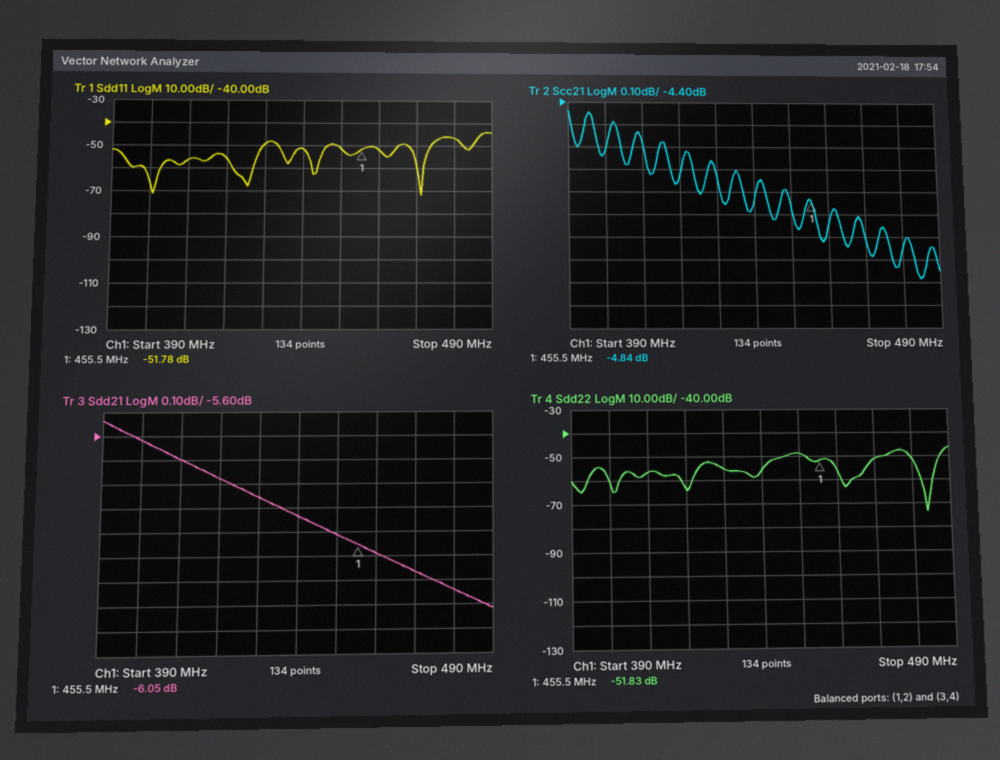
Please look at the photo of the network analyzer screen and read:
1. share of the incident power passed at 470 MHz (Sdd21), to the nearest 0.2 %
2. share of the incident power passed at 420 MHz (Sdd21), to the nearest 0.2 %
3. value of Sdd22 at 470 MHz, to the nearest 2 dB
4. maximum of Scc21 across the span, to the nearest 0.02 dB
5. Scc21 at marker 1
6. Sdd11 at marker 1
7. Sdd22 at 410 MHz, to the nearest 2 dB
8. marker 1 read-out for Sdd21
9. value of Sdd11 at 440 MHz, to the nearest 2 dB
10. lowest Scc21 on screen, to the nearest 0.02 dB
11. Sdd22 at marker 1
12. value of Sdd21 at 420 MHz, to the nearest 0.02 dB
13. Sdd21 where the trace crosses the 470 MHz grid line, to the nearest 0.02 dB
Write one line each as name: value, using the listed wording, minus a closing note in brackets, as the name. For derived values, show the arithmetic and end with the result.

share of the incident power passed at 470 MHz (Sdd21), to the nearest 0.2 %: 10^(-6.16/10) ≈ 24.2 %
share of the incident power passed at 420 MHz (Sdd21), to the nearest 0.2 %: 10^(-5.78/10) ≈ 26.4 %
value of Sdd22 at 470 MHz, to the nearest 2 dB: -52 dB
maximum of Scc21 across the span, to the nearest 0.02 dB: -4.44 dB
Scc21 at marker 1: -4.84 dB
Sdd11 at marker 1: -51.78 dB
Sdd22 at 410 MHz, to the nearest 2 dB: -56 dB
marker 1 read-out for Sdd21: -6.05 dB
value of Sdd11 at 440 MHz, to the nearest 2 dB: -52 dB
lowest Scc21 on screen, to the nearest 0.02 dB: -5.18 dB
Sdd22 at marker 1: -51.83 dB
value of Sdd21 at 420 MHz, to the nearest 0.02 dB: -5.78 dB
Sdd21 where the trace crosses the 470 MHz grid line, to the nearest 0.02 dB: -6.16 dB
